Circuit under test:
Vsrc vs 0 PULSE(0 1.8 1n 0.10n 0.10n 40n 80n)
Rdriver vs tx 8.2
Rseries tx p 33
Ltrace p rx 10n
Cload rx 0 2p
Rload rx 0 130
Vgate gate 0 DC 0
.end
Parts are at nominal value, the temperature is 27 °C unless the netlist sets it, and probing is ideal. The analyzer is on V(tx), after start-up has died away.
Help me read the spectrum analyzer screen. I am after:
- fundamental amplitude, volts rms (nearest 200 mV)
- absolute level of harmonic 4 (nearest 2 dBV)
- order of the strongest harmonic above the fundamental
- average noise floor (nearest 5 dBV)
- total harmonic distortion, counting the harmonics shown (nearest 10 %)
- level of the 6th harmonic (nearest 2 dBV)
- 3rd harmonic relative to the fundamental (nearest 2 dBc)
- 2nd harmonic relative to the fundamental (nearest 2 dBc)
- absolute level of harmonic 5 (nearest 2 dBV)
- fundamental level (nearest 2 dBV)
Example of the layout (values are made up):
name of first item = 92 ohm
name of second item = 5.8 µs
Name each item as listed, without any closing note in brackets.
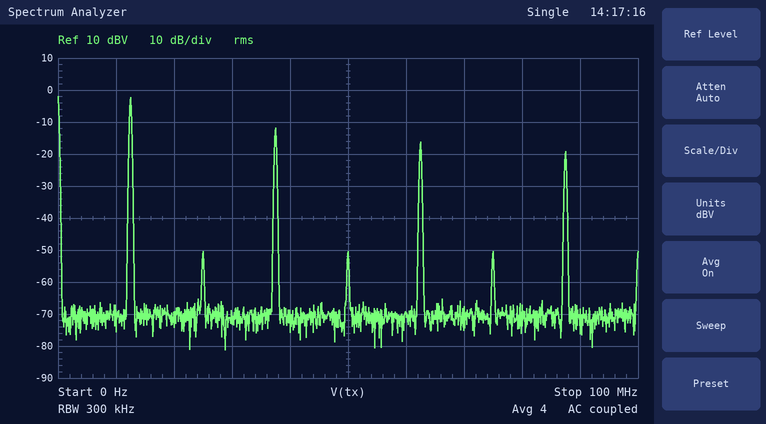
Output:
fundamental amplitude, volts rms = 800 mV
absolute level of harmonic 4 = -50 dBV
order of the strongest harmonic above the fundamental = 3
average noise floor = -70 dBV
total harmonic distortion, counting the harmonics shown = 40 %
level of the 6th harmonic = -50 dBV
3rd harmonic relative to the fundamental = -10 dBc
2nd harmonic relative to the fundamental = -48 dBc
absolute level of harmonic 5 = -16 dBV
fundamental level = -2 dBV
